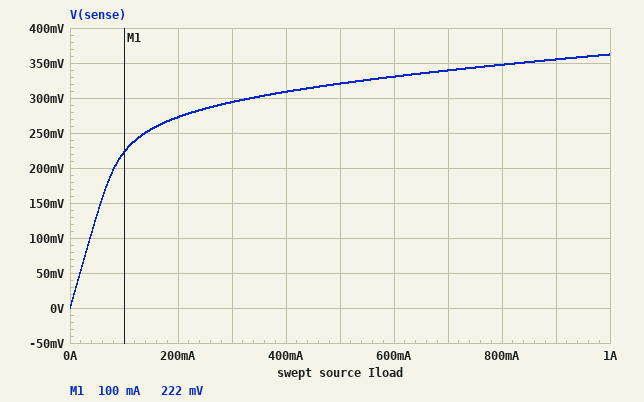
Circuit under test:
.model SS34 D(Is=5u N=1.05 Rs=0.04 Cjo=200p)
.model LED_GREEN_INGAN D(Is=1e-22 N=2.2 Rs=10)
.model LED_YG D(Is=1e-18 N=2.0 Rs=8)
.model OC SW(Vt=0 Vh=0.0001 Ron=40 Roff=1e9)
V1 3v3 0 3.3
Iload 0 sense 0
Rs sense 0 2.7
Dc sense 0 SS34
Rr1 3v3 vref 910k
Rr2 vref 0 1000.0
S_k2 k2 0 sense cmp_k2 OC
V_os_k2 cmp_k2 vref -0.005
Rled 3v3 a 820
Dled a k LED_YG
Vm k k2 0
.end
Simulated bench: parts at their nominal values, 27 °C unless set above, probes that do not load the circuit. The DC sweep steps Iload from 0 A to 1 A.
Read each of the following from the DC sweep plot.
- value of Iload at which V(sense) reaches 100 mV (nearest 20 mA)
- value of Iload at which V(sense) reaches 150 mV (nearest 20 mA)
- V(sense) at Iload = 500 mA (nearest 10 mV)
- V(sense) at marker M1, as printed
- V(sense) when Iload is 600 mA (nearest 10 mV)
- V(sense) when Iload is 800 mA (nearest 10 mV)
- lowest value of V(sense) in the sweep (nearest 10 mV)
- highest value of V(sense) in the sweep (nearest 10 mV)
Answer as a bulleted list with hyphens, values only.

- 40 mA
- 60 mA
- 320 mV
- 222 mV
- 330 mV
- 350 mV
- 0 V
- 360 mV
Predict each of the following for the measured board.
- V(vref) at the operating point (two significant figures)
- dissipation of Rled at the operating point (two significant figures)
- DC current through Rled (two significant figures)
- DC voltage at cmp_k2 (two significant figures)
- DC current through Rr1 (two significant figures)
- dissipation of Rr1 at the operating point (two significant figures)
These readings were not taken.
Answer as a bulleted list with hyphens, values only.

- 3.6 mV
- 2.4 mW
- 1.7 mA
- -1.4 mV
- 3.6 µA
- 12 µW
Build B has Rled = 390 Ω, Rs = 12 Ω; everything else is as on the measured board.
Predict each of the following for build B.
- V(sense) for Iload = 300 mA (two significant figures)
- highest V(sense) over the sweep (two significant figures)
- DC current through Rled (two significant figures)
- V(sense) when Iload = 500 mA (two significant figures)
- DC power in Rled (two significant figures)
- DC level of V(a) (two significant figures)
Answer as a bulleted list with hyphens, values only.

- 310 mV
- 370 mV
- 3.3 mA
- 330 mV
- 4.3 mW
- 2.0 V
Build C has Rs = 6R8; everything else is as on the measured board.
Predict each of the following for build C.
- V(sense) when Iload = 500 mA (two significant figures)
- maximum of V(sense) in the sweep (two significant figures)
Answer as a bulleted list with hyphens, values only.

- 330 mV
- 370 mV
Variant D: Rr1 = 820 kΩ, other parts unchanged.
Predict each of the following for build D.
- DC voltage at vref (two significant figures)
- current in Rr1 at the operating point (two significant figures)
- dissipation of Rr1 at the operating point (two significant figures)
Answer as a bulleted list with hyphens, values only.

- 4.0 mV
- 4.0 µA
- 13 µW
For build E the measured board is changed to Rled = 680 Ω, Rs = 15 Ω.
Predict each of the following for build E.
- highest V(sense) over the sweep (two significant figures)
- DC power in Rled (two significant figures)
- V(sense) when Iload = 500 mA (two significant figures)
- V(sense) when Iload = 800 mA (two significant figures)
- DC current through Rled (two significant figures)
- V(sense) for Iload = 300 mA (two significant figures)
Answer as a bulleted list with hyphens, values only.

- 370 mV
- 2.8 mW
- 330 mV
- 360 mV
- 2.0 mA
- 310 mV
